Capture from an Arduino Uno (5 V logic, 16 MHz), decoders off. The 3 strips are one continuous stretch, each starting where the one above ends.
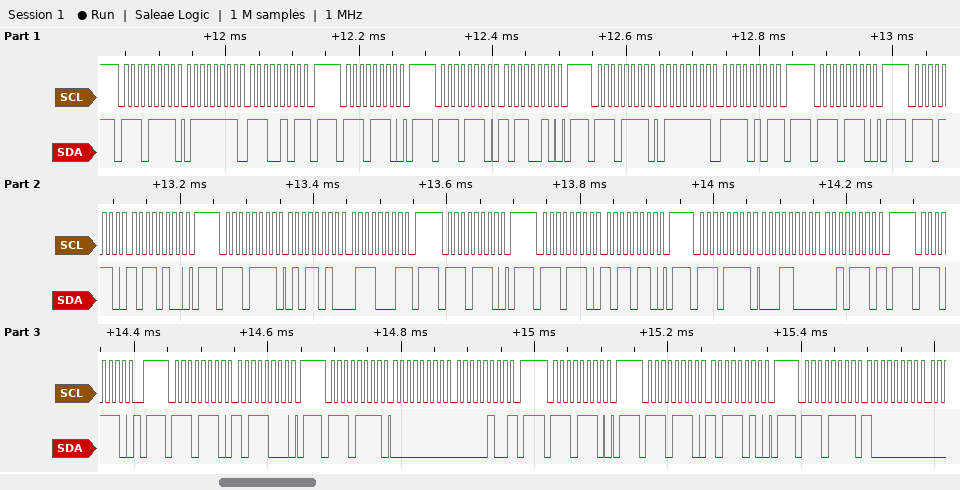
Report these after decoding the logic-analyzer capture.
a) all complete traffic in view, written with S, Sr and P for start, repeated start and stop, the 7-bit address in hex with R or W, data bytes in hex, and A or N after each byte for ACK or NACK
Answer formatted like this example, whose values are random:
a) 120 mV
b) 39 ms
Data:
a) S 77R A 7F A E5 N P S 77W A P S 77W A B2 A P S 77R A 7F A F5 N P S 77W A P S 77W A B4 A P S 77R A 5A A 71 N P S 77W A P S 77W A B6 A P S 77R A 18 A 2E N P S 77W A P S 77W A B8 A P S 77R A 00 A 04 N P S 77W A P S 77W A BA A P S 77R A 80 A
